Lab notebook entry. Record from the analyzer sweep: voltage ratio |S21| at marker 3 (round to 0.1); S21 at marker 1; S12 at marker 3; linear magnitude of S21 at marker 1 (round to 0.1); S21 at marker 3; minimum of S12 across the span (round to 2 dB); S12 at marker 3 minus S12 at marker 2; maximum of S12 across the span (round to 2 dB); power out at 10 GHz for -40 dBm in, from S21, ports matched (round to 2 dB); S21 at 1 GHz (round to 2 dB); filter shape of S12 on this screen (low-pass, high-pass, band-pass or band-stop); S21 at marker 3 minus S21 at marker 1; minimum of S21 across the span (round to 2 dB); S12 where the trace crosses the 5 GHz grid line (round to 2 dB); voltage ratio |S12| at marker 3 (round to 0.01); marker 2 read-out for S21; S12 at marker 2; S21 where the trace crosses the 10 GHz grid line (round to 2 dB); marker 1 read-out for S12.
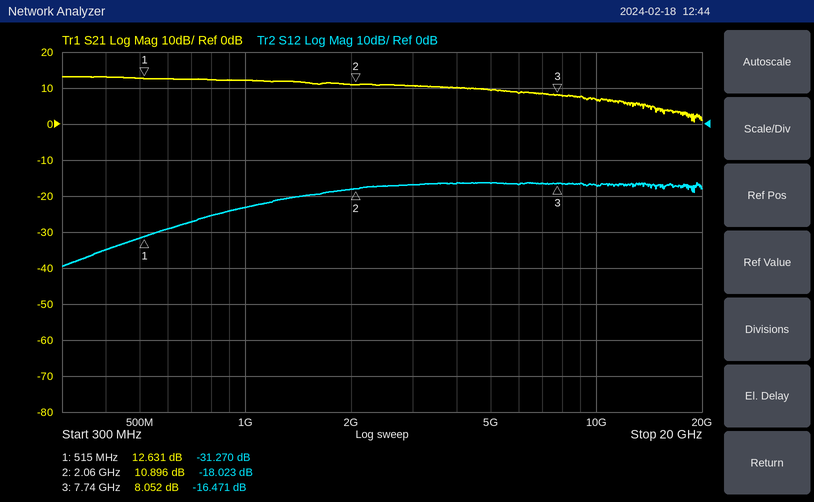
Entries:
2.5
12.631 dB
-16.471 dB
4.3
8.052 dB
-40 dB
1.552 dB
-16 dB
-34 dBm
12 dB
high-pass
-4.579 dB
0 dB
-16 dB
0.15
10.896 dB
-18.023 dB
6 dB
-31.270 dB
